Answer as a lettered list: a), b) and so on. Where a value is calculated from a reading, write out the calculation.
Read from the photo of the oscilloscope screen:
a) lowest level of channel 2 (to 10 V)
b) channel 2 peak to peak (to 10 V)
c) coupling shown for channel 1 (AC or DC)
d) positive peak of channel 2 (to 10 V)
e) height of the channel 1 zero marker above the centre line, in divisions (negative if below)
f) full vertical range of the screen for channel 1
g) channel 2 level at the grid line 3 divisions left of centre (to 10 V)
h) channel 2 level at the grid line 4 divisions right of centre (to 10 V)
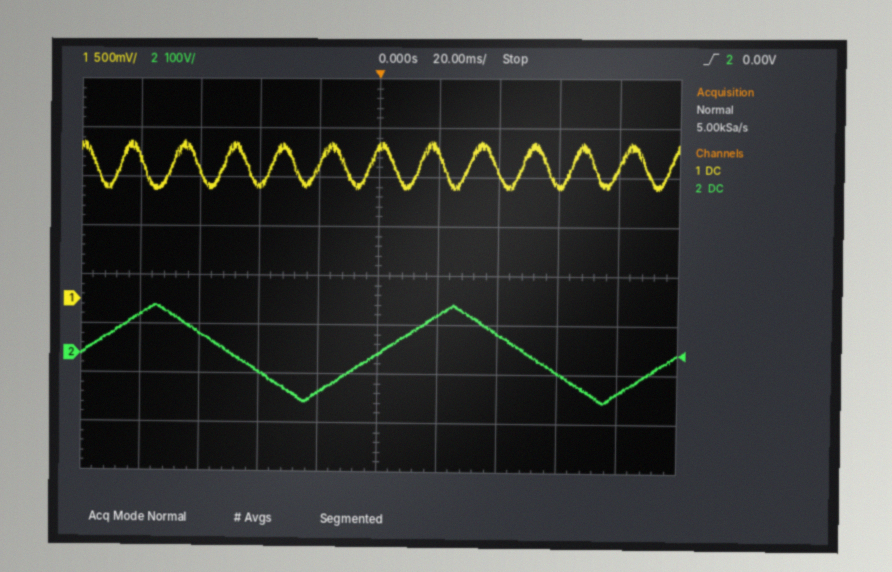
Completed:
a) -100 V
b) 100 V − (-100 V) = 200 V
c) DC
d) 100 V
e) -0.5 div
f) 4 V
g) 40 V
h) -80 V
